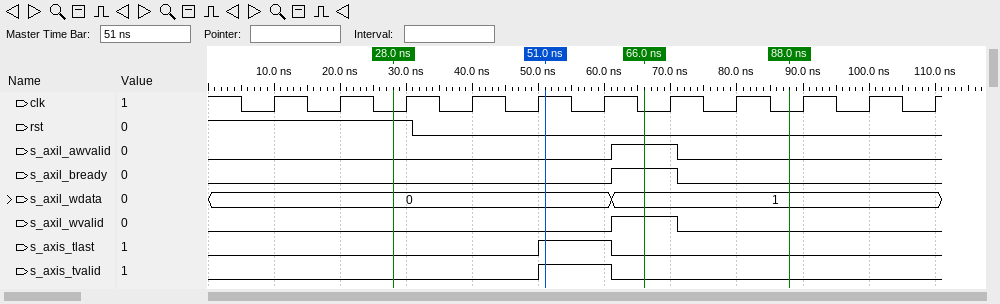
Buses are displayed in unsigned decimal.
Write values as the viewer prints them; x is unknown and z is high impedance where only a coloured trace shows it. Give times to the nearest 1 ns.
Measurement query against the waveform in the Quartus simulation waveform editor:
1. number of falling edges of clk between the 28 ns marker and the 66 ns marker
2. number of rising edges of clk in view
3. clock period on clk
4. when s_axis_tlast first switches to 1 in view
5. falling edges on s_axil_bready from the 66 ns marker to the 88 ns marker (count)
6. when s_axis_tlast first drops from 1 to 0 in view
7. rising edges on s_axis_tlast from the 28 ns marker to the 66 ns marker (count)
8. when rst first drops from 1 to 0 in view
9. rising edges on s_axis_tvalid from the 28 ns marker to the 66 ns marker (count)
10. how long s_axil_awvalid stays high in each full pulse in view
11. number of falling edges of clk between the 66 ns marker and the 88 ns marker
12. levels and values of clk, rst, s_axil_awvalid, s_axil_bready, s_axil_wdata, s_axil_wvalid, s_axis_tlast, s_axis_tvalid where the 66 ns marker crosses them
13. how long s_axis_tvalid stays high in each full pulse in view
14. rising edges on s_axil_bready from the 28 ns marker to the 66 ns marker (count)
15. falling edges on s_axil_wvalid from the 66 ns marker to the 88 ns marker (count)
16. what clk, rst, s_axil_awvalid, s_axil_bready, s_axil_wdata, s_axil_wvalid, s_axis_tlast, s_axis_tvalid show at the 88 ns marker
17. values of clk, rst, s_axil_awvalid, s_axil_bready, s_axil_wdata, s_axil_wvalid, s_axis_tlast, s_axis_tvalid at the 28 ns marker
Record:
4
11
10 ns
50 ns
1
61 ns
1
31 ns
1
10 ns
2
clk=0, rst=0, s_axil_awvalid=1, s_axil_bready=1, s_axil_wdata=1, s_axil_wvalid=1, s_axis_tlast=0, s_axis_tvalid=0
11 ns
1
1
clk=0, rst=0, s_axil_awvalid=0, s_axil_bready=0, s_axil_wdata=1, s_axil_wvalid=0, s_axis_tlast=0, s_axis_tvalid=0
clk=0, rst=1, s_axil_awvalid=0, s_axil_bready=0, s_axil_wdata=0, s_axil_wvalid=0, s_axis_tlast=0, s_axis_tvalid=0
